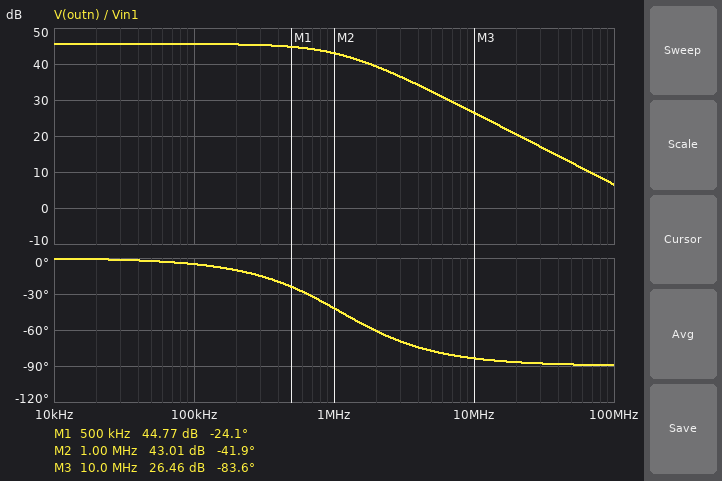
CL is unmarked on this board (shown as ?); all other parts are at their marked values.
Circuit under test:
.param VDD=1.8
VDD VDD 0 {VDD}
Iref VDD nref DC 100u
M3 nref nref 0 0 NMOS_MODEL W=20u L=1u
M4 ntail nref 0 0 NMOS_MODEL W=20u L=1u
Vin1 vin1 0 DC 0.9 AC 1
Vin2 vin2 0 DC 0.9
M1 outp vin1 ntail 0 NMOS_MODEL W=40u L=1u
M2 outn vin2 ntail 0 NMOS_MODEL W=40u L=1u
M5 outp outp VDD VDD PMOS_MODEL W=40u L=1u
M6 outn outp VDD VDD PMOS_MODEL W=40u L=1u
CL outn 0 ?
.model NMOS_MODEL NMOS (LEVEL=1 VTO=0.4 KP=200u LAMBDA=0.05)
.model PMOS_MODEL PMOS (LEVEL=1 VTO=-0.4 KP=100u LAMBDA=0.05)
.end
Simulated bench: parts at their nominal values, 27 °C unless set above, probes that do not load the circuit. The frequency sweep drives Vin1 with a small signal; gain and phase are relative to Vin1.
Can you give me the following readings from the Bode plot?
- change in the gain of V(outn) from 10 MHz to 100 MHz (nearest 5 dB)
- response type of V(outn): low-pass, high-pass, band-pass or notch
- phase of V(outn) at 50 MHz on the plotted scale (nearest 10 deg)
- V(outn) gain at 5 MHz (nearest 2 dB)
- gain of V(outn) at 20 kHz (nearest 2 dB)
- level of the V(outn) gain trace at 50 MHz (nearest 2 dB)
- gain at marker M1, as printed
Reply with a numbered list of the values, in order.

1. -20 dB
2. low-pass
3. -90 deg
4. 32 dB
5. 46 dB
6. 12 dB
7. 44.77 dB
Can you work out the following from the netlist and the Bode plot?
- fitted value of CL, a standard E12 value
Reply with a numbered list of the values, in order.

1. 680 fF
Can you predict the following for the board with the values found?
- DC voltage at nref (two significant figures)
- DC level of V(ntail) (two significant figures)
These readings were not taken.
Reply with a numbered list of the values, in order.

1. 620 mV
2. 390 mV
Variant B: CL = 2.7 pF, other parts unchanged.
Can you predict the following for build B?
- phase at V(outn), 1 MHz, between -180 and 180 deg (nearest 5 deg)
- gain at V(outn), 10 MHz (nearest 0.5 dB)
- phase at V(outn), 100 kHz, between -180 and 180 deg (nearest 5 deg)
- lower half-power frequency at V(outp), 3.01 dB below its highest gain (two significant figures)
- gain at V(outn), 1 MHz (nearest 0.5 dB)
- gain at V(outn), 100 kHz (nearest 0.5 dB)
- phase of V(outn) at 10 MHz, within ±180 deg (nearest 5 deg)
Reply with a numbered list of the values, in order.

1. -75 deg
2. 14.5 dB
3. -20 deg
4. 200 kHz
5. 34.0 dB
6. 45.0 dB
7. -90 deg
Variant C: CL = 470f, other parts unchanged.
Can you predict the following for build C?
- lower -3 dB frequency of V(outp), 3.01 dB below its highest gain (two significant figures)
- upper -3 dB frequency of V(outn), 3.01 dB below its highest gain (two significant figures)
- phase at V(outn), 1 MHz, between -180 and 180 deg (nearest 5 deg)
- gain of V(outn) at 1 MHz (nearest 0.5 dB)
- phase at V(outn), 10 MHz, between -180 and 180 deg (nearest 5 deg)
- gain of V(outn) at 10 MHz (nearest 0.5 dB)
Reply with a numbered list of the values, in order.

1. 1.1 MHz
2. 1.6 MHz
3. -30 deg
4. 44.0 dB
5. -80 deg
6. 29.5 dB
